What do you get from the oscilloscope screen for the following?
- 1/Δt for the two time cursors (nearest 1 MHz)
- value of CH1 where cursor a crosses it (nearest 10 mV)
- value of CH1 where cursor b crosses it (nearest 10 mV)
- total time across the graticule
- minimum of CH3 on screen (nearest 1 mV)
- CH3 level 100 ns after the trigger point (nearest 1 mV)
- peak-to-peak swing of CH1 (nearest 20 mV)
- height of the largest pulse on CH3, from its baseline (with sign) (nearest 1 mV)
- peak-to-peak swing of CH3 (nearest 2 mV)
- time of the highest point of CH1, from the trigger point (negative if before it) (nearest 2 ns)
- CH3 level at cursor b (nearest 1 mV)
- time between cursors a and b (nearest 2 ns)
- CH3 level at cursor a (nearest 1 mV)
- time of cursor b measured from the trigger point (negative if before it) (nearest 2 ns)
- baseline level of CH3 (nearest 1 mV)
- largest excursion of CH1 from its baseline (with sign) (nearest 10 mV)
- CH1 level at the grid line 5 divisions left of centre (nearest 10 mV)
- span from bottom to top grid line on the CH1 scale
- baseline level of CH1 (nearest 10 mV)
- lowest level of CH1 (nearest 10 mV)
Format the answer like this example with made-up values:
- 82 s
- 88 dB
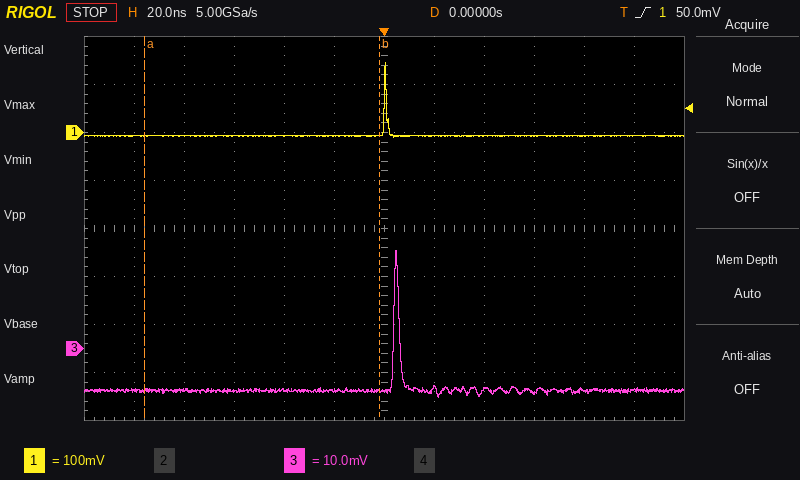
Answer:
- 11 MHz
- -10 mV
- 0 mV
- 240 ns
- -10 mV
- -9 mV
- 160 mV
- +29 mV
- 30 mV
- 0 ns
- -9 mV
- 94 ns
- -9 mV
- -2 ns
- -9 mV
- +150 mV
- -10 mV
- 800 mV
- -10 mV
- -10 mV
